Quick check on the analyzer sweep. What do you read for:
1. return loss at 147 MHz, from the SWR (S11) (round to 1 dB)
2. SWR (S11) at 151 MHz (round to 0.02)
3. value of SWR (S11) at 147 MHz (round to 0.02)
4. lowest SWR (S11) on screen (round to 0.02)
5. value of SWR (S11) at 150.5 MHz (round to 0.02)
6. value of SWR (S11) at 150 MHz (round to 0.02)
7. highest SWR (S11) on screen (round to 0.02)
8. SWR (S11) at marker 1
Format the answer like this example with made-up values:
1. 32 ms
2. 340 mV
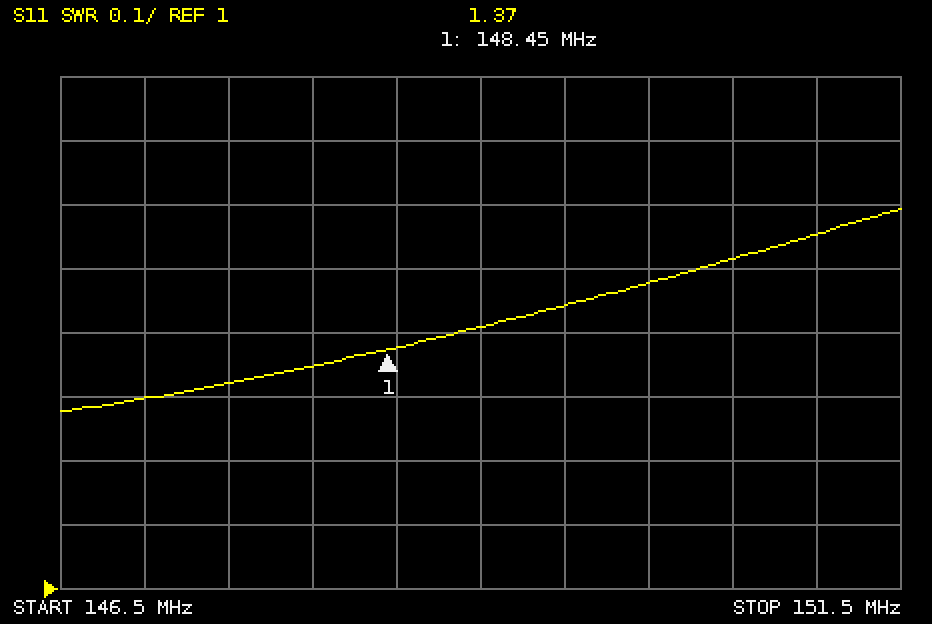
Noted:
1. 18 dB
2. 1.56
3. 1.30
4. 1.28
5. 1.52
6. 1.48
7. 1.60
8. 1.37
